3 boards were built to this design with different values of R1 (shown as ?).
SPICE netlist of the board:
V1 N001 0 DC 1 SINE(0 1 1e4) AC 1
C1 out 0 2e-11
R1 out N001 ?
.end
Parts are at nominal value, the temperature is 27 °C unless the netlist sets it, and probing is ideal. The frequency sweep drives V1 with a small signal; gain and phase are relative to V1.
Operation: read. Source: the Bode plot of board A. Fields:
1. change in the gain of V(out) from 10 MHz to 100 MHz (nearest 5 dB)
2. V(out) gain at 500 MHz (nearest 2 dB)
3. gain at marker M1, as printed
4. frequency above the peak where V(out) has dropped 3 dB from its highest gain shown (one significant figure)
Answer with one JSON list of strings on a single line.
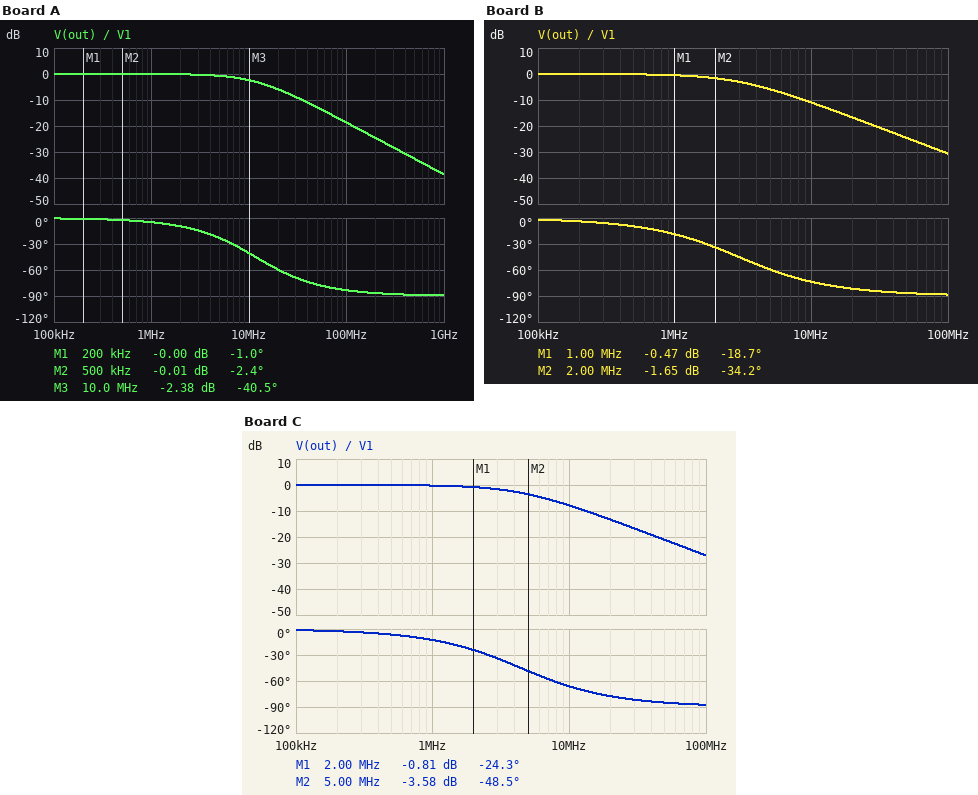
["-15 dB", "-32 dB", "-0.00 dB", "10 MHz"]
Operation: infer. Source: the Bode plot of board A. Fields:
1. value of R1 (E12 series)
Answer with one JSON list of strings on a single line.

["680 Ω"]
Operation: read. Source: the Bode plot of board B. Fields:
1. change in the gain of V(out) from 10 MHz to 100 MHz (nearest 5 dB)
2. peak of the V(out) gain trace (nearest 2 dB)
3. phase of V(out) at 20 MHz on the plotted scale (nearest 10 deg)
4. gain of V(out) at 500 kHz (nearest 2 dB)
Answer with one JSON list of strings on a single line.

["-20 dB", "0 dB", "-80 deg", "0 dB"]
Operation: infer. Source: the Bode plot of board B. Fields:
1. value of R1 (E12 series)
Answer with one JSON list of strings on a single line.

["2.7 kΩ"]
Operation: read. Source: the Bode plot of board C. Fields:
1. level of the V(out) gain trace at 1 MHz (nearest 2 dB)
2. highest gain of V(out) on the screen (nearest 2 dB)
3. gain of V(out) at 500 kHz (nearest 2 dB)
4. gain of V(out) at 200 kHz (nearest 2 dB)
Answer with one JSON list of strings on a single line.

["0 dB", "0 dB", "0 dB", "0 dB"]
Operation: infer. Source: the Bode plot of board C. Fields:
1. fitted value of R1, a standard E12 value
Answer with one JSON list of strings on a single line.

["1.8 kΩ"]
